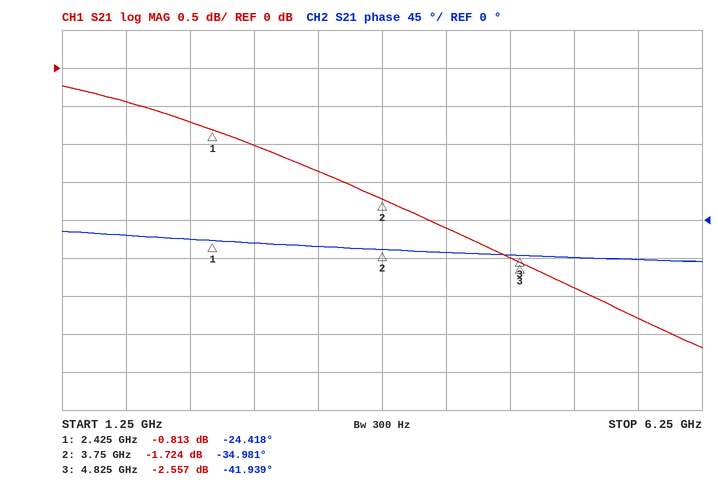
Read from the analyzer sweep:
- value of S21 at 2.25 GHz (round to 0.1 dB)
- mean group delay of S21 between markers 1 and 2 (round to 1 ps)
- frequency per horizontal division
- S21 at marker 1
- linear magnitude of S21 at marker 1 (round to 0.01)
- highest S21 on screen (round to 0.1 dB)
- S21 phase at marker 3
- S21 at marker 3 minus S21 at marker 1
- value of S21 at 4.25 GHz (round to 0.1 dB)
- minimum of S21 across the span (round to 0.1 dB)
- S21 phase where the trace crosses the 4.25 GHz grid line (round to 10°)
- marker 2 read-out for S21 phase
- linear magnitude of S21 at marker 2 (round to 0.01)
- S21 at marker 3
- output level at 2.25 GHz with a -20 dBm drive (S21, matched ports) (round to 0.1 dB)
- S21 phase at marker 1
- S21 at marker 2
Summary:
-0.7 dB
22 ps
500 MHz
-0.813 dB
0.91
-0.2 dB
-41.939°
-1.744 dB
-2.1 dB
-3.7 dB
-40°
-34.981°
0.82
-2.557 dB
-20.7 dBm
-24.418°
-1.724 dB
